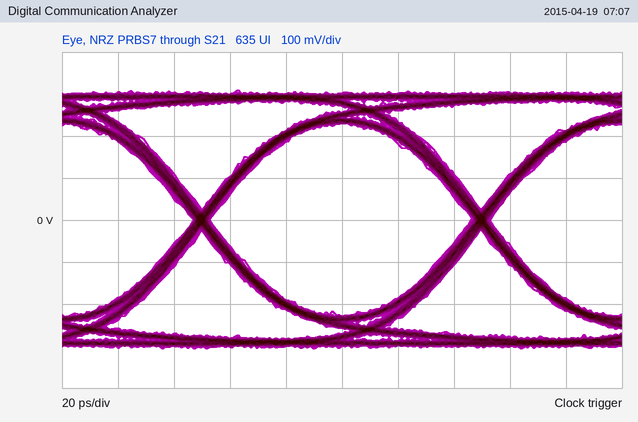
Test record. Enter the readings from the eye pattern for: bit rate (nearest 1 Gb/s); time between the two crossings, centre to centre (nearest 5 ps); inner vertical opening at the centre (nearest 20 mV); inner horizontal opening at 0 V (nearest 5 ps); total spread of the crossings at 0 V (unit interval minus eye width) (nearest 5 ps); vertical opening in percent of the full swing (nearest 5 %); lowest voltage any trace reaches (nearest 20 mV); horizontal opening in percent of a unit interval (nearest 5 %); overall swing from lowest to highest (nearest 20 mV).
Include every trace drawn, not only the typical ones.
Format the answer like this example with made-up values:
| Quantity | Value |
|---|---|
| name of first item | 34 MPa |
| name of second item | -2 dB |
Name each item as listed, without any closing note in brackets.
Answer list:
| Quantity | Value |
|---|---|
| bit rate | 10 Gb/s |
| time between the two crossings, centre to centre | 100 ps |
| inner vertical opening at the centre | 460 mV |
| inner horizontal opening at 0 V | 95 ps |
| total spread of the crossings at 0 V (unit interval minus eye width) | 5 ps |
| vertical opening in percent of the full swing | 75 % |
| lowest voltage any trace reaches | -300 mV |
| horizontal opening in percent of a unit interval | 95 % |
| overall swing from lowest to highest | 620 mV |
